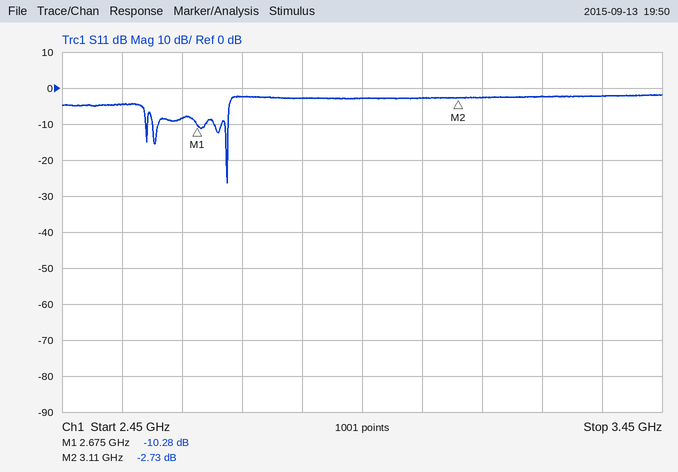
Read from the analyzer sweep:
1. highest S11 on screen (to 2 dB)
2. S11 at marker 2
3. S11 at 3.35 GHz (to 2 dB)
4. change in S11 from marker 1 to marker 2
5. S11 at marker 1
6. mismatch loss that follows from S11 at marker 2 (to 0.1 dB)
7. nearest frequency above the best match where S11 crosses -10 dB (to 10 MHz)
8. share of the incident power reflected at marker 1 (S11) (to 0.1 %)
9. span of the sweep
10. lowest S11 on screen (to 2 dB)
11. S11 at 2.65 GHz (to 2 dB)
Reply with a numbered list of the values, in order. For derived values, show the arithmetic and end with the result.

1. -2 dB
2. -2.73 dB
3. -2 dB
4. -2.73 − (-10.28) = 7.55 dB
5. -10.28 dB
6. −10 log10(1 − 10^(-2.73/10)) ≈ 3.3 dB
7. 2.73 GHz
8. 10^(-10.28/10) ≈ 9.4 %
9. 1 GHz
10. -26 dB
11. -8 dB
